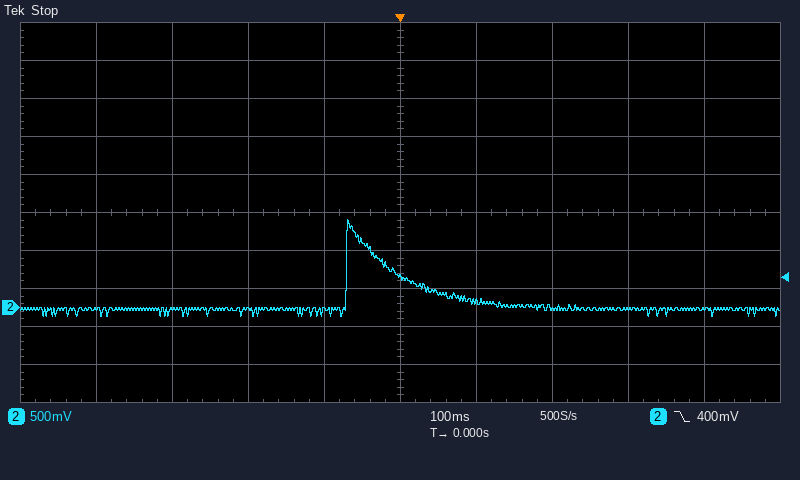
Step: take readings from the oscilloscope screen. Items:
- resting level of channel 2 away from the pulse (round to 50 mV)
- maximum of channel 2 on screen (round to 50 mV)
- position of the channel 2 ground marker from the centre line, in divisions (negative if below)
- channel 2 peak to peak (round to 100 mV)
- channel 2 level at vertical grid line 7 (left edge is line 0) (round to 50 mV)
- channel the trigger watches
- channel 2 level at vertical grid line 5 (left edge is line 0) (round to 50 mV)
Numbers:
0 mV
1.15 V
-2.5 div
1.30 V
0 mV
channel 2
400 mV
